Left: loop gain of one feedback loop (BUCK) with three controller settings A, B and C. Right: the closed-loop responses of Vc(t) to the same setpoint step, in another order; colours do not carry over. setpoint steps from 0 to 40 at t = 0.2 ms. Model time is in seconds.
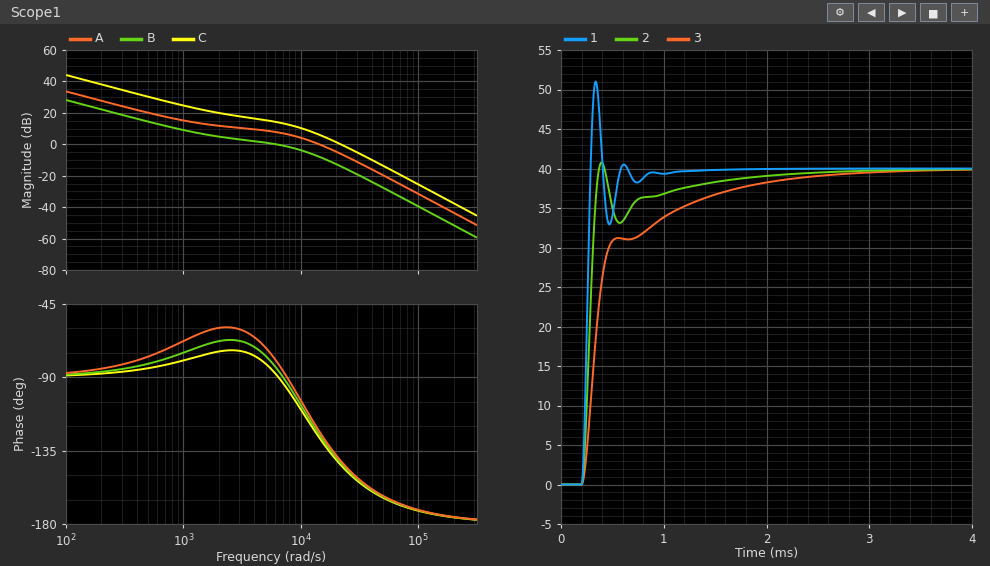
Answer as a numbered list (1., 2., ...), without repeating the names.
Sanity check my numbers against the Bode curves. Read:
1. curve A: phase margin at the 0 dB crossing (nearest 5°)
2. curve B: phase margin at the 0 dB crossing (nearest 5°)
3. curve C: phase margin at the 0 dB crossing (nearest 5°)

1. 55°
2. 95°
3. 35°
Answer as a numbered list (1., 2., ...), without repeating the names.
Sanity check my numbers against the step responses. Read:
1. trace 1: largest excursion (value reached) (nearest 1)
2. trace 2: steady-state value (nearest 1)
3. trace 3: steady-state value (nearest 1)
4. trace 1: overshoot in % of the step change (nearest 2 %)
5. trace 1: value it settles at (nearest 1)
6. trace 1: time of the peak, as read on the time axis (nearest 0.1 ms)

1. 51
2. 40
3. 40
4. 28 %
5. 40
6. 0.3 ms
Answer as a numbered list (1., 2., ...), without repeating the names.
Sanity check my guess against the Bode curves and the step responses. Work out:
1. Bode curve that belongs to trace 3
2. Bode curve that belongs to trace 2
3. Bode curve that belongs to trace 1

1. B
2. A
3. C
